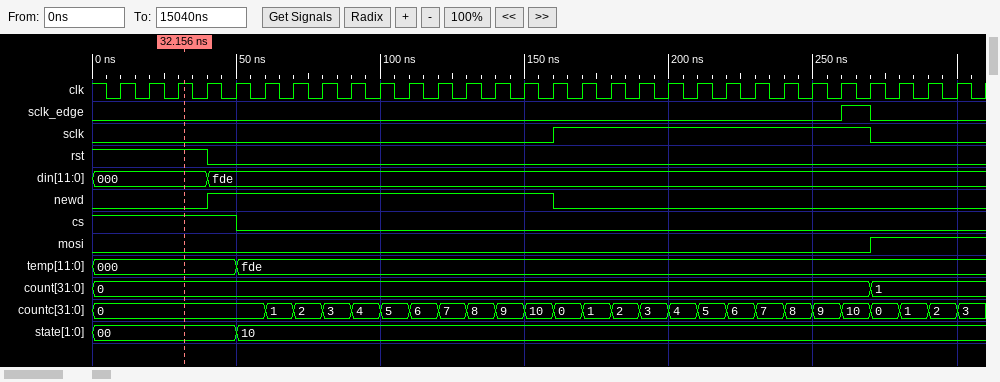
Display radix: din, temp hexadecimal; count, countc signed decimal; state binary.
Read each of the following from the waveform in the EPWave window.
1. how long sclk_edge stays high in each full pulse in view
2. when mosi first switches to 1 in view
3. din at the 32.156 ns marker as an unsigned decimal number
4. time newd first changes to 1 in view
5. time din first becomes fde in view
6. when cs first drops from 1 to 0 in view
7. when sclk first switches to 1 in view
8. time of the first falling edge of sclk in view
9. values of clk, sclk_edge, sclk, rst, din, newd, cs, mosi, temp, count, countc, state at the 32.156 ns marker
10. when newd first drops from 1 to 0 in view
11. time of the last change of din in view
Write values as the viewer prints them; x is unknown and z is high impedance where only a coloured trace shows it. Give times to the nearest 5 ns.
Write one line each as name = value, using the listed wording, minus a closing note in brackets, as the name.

how long sclk_edge stays high in each full pulse in view = 10 ns
when mosi first switches to 1 in view = 270 ns
din at the 32.156 ns marker as an unsigned decimal number = 0
time newd first changes to 1 in view = 40 ns
time din first becomes fde in view = 40 ns
when cs first drops from 1 to 0 in view = 50 ns
when sclk first switches to 1 in view = 160 ns
time of the first falling edge of sclk in view = 270 ns
values of clk, sclk_edge, sclk, rst, din, newd, cs, mosi, temp, count, countc, state at the 32.156 ns marker = clk=1, sclk_edge=0, sclk=0, rst=1, din=000, newd=0, cs=1, mosi=0, temp=000, count=0, countc=0, state=00
when newd first drops from 1 to 0 in view = 160 ns
time of the last change of din in view = 40 ns
